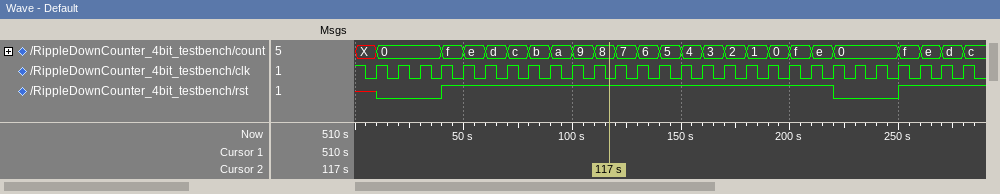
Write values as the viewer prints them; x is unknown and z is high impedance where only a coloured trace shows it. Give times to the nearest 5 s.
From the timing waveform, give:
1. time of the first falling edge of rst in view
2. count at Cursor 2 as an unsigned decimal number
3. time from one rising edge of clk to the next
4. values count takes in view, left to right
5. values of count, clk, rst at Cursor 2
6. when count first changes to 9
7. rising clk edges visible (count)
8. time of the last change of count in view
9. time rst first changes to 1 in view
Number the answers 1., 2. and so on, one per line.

1. 220 s
2. 8
3. 10 s
4. X, 0, f, e, d, c, b, a, 9, 8, 7, 6, 5, 4, 3, 2, 1, 0, f, e, 0, f, e, d, c
5. count=8, clk=0, rst=1
6. 100 s
7. 28
8. 280 s
9. 40 s
